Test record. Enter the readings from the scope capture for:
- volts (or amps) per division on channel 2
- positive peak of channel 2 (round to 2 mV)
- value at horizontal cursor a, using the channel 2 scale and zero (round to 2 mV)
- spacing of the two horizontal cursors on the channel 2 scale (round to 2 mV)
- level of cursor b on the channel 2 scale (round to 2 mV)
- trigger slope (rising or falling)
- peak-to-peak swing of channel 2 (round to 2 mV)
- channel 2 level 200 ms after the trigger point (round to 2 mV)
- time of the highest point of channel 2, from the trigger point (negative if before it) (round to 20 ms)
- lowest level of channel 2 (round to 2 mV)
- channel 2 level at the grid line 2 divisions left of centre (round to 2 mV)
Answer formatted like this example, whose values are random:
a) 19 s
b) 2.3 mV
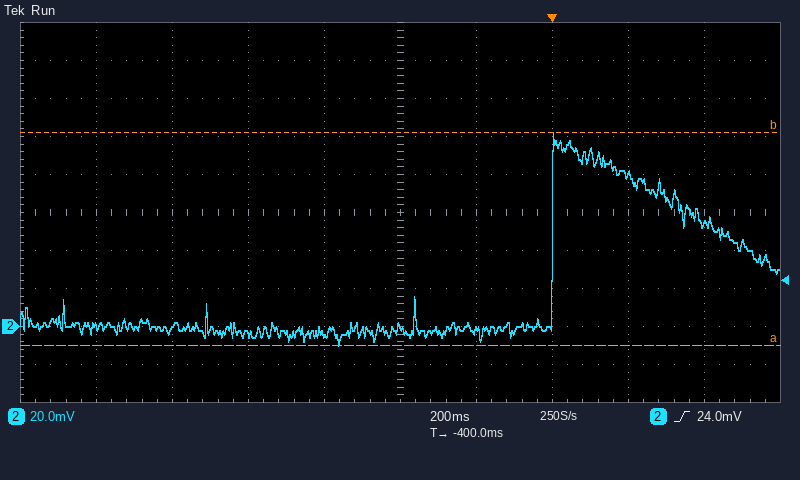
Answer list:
a) 20 mV
b) 102 mV
c) -10 mV
d) 112 mV
e) 102 mV
f) rising
g) 112 mV
h) 80 mV
i) 0 ms
j) -10 mV
k) -4 mV
